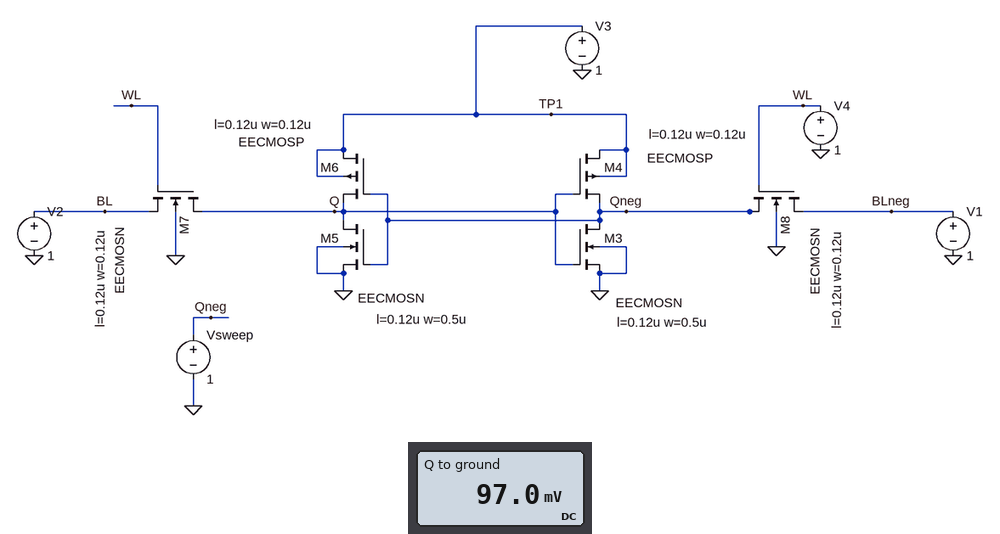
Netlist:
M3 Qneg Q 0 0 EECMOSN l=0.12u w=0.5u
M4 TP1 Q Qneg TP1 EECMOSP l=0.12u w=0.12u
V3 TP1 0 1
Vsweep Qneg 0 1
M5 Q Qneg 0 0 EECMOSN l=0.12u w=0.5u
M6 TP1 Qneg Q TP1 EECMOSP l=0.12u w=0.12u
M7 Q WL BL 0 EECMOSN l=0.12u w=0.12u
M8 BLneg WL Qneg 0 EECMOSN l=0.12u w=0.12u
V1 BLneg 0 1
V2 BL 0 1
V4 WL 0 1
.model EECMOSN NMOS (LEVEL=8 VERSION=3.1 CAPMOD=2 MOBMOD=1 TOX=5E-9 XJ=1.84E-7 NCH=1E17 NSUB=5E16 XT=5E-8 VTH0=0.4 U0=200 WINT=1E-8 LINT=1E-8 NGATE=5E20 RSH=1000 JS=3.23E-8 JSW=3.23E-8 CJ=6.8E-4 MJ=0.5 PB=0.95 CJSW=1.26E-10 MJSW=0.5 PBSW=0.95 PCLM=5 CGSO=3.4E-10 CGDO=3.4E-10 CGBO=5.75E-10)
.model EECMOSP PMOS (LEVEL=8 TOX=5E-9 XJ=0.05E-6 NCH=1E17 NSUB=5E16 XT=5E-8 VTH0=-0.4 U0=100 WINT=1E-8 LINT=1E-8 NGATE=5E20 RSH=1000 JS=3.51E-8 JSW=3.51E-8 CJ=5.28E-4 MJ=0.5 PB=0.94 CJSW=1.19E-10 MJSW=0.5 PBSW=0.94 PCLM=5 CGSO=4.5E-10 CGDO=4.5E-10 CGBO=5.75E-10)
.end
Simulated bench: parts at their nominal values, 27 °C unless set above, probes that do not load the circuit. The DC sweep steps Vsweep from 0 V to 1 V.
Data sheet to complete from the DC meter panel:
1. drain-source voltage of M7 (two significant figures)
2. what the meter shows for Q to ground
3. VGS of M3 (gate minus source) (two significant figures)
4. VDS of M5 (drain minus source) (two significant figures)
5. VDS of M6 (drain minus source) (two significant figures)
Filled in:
-900 mV
97.0 mV
97 mV
97 mV
900 mV
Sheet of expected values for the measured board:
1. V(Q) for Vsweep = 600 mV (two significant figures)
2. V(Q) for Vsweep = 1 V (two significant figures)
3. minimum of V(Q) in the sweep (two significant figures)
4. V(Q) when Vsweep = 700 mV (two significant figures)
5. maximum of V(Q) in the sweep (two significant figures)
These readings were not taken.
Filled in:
170 mV
97 mV
97 mV
130 mV
1.0 V
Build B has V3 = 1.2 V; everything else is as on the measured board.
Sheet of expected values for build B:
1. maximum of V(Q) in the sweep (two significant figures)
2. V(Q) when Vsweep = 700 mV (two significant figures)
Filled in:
1.2 V
150 mV
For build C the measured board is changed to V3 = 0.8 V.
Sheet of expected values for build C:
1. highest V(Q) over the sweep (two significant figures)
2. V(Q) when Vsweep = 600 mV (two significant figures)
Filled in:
800 mV
160 mV
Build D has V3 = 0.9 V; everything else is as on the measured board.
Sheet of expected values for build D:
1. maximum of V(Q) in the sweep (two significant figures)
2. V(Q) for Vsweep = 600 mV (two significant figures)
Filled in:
900 mV
160 mV
